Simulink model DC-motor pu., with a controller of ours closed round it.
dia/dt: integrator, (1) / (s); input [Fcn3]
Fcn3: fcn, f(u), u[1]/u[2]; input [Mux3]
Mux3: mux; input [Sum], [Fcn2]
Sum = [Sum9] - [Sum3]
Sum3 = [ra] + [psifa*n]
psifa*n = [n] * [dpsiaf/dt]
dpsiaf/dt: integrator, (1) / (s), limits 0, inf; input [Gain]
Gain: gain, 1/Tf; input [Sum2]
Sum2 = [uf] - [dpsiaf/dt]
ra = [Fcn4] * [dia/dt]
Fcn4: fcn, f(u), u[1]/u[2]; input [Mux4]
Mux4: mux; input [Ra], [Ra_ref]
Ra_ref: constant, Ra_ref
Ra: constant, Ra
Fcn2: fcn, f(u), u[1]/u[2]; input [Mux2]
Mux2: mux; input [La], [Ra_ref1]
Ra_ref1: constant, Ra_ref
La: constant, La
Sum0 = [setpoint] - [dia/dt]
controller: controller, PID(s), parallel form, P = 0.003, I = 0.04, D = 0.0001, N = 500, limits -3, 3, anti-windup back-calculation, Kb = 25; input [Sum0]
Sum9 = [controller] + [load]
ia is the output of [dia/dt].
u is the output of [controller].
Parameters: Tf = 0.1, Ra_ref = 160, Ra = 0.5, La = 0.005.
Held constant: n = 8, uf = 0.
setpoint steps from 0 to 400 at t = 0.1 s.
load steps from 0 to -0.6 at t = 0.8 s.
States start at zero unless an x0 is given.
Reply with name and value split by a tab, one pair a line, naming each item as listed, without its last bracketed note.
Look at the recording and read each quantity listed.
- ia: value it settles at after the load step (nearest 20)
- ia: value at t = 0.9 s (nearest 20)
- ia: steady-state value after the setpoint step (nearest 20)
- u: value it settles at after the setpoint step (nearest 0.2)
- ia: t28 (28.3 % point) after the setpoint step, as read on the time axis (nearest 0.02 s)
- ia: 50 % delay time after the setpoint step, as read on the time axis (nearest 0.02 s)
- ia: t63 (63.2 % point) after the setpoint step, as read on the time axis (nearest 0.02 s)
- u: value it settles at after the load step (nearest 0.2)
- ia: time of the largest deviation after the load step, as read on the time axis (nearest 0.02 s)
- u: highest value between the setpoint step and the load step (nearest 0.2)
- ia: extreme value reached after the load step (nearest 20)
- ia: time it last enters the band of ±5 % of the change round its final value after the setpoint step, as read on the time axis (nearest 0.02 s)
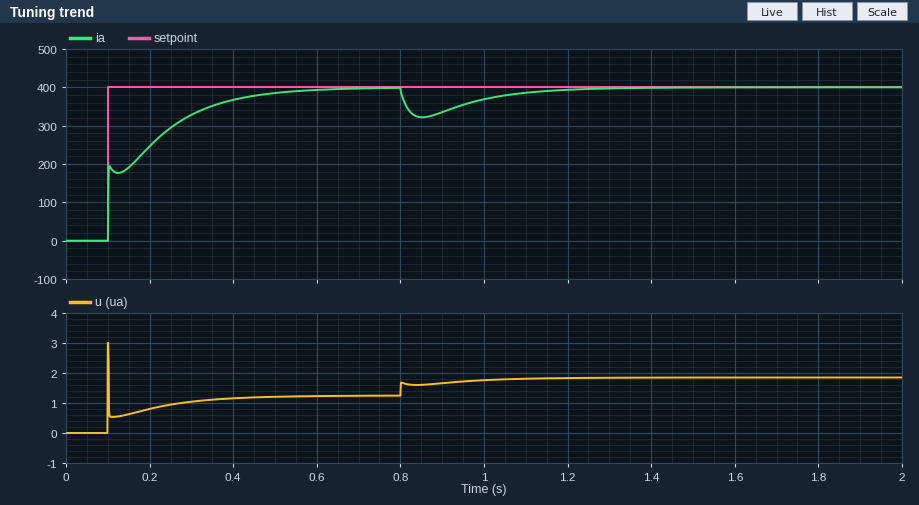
ia: value it settles at after the load step	400
ia: value at t = 0.9 s	340
ia: steady-state value after the setpoint step	400
u: value it settles at after the setpoint step	1.2
ia: t28 (28.3 % point) after the setpoint step, as read on the time axis	0.10 s
ia: 50 % delay time after the setpoint step, as read on the time axis	0.16 s
ia: t63 (63.2 % point) after the setpoint step, as read on the time axis	0.20 s
u: value it settles at after the load step	1.8
ia: time of the largest deviation after the load step, as read on the time axis	0.86 s
u: highest value between the setpoint step and the load step	3.0
ia: extreme value reached after the load step	320
ia: time it last enters the band of ±5 % of the change round its final value after the setpoint step, as read on the time axis	0.46 s
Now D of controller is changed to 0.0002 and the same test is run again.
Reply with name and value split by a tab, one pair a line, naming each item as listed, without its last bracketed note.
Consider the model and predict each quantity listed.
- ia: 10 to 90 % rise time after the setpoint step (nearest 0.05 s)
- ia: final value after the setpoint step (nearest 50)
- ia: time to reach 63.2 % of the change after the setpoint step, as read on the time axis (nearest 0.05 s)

ia: 10 to 90 % rise time after the setpoint step	0.30 s
ia: final value after the setpoint step	400
ia: time to reach 63.2 % of the change after the setpoint step, as read on the time axis	0.25 s
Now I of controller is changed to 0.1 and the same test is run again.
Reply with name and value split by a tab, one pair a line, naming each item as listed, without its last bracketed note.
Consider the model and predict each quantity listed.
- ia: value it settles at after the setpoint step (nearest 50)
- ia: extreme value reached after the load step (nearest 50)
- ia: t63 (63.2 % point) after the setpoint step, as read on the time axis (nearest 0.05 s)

ia: value it settles at after the setpoint step	400
ia: extreme value reached after the load step	350
ia: t63 (63.2 % point) after the setpoint step, as read on the time axis	0.15 s
